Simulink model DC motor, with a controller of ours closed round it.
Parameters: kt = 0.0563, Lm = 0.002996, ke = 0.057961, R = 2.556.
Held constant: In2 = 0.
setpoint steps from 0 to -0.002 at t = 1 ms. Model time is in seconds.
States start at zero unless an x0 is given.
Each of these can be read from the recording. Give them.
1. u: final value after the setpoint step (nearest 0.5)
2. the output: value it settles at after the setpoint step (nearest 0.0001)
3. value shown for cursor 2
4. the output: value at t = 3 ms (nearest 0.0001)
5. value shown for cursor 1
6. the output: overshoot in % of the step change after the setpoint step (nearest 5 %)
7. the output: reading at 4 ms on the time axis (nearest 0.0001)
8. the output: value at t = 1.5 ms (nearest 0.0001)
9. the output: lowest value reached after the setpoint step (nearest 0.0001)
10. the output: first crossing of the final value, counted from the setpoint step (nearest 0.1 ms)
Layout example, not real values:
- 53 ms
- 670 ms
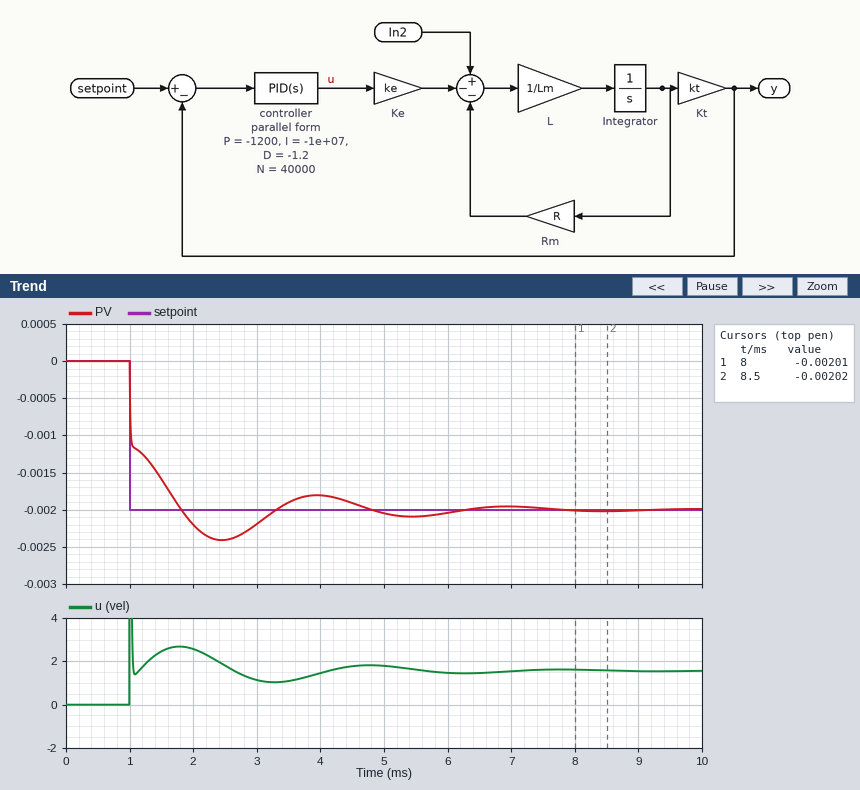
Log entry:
- 1.5
- -0.0020
- -0.00202
- -0.0022
- -0.00201
- 20 %
- -0.0018
- -0.0016
- -0.0024
- 0.8 ms
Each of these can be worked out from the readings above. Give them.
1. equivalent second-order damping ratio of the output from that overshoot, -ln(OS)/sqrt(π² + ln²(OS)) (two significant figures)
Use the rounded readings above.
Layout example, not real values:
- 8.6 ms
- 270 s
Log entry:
- 0.46
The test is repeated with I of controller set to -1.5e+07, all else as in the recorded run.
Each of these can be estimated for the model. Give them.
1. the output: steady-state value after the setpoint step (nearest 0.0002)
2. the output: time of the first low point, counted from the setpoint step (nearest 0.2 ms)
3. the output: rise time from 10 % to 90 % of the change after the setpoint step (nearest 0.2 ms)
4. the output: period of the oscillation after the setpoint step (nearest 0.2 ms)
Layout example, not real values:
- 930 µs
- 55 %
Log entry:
- -0.0020
- 1.2 ms
- 0.6 ms
- 2.4 ms
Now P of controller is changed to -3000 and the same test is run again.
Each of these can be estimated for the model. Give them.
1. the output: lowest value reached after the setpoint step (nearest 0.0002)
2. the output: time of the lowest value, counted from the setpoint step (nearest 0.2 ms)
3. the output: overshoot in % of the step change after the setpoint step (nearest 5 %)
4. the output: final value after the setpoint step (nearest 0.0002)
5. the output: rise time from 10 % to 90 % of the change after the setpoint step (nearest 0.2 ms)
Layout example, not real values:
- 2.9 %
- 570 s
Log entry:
- -0.0022
- 1.4 ms
- 10 %
- -0.0020
- 0.6 ms
